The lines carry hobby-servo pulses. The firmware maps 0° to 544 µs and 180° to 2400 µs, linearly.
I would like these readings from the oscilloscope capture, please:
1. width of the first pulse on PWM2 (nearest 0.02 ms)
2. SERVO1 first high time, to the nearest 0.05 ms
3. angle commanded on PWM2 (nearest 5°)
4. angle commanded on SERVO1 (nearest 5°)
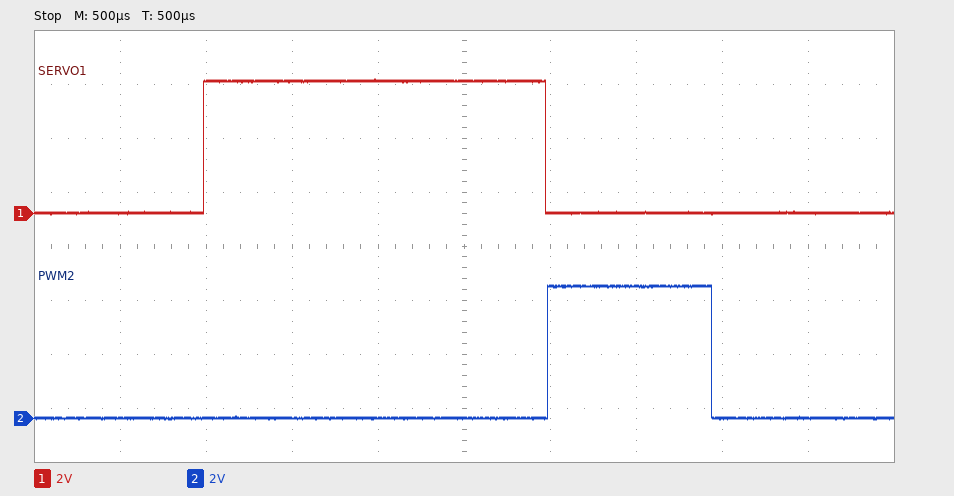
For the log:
0.96 ms
2.00 ms
40°
140°
